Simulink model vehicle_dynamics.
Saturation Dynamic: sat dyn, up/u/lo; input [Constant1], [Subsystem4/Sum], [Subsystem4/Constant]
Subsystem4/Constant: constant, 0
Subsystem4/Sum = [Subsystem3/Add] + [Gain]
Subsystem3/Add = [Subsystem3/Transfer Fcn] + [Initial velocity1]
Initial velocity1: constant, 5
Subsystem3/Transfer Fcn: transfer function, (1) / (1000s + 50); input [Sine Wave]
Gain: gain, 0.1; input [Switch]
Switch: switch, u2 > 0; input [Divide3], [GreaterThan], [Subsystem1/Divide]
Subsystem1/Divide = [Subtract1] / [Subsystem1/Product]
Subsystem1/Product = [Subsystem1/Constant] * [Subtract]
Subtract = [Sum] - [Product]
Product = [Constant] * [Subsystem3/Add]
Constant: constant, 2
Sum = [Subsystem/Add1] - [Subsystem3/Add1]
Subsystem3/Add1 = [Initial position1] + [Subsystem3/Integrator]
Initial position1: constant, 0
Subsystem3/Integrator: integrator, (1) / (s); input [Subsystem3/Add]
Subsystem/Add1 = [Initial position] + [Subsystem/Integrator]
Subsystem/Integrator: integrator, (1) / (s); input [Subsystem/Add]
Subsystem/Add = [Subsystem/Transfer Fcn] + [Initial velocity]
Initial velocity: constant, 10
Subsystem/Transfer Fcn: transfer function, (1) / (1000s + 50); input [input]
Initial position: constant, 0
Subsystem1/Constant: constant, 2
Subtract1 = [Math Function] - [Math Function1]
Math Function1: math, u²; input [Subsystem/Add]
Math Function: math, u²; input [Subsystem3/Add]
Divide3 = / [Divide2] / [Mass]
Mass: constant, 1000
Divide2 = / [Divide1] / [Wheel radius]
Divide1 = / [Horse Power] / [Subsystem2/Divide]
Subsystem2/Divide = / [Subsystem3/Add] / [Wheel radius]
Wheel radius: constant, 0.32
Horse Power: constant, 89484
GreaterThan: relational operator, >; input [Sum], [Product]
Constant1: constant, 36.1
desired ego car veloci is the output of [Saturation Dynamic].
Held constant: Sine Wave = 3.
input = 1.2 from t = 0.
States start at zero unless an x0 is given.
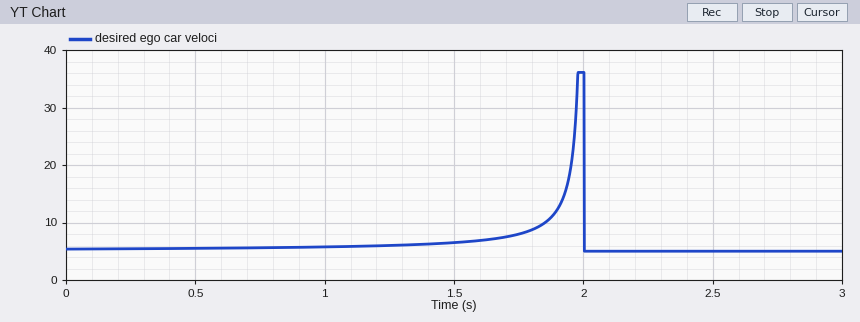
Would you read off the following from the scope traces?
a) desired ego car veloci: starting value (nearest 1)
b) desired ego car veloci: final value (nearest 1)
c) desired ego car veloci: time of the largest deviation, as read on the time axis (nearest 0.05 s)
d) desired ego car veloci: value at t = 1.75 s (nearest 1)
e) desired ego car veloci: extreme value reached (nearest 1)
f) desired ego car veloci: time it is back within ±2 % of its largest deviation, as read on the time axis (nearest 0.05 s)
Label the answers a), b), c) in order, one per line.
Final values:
a) 5
b) 5
c) 2.00 s
d) 8
e) 36
f) 2.00 s
